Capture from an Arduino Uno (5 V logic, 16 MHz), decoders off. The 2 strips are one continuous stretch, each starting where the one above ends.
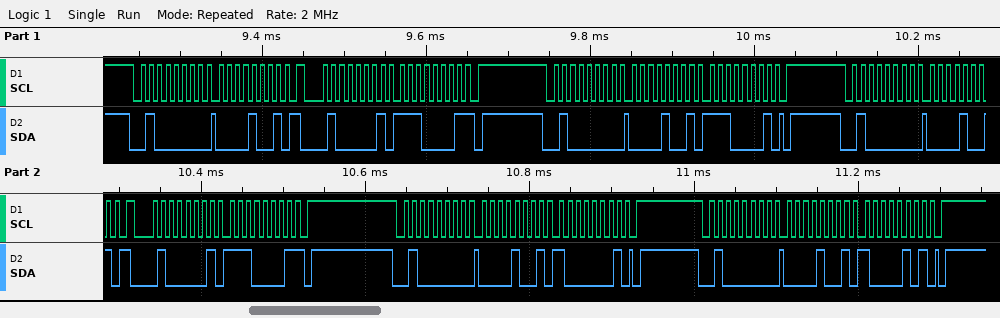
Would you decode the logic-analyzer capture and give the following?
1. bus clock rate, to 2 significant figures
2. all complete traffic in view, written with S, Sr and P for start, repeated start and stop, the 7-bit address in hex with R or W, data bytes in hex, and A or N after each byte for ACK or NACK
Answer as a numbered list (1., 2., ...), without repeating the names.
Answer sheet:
1. 100 kHz
2. S 20W A 09 A Sr 20R A E1 N P S 20W A 09 A E1 A P S 20W A 09 A Sr 20R A E1 N P S 20W A 09 A 81 A P S 20W A 09 A 85 A P
